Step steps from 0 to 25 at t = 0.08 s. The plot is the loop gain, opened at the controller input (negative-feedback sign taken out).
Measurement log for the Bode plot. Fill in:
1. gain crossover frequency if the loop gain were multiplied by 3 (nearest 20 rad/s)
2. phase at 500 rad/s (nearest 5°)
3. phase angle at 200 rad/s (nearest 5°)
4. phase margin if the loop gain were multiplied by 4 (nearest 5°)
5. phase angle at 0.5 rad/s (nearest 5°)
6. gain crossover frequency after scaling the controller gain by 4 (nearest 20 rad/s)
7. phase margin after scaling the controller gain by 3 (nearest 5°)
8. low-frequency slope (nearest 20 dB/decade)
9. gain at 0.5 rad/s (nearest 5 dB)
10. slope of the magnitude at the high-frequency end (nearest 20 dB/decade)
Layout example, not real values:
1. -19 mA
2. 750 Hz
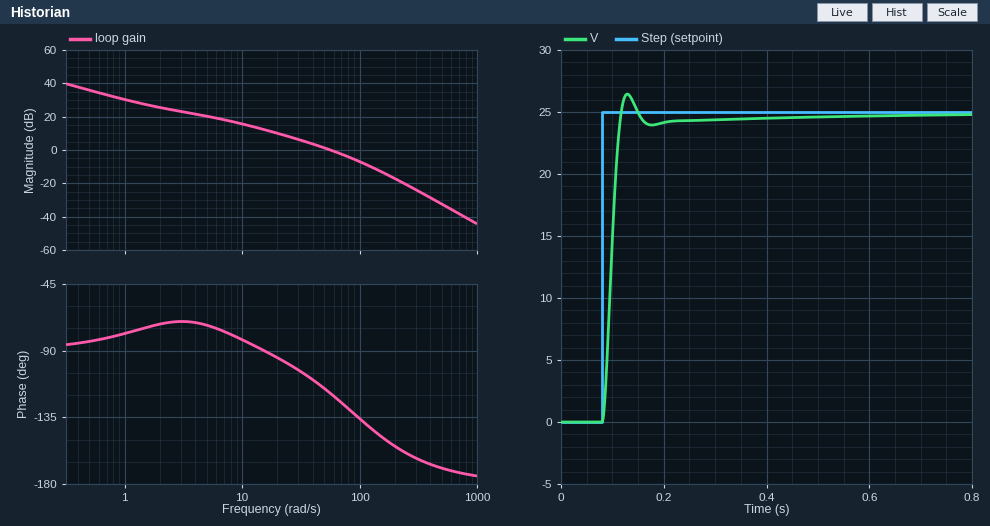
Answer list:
1. 120 rad/s
2. -170°
3. -155°
4. 35°
5. -85°
6. 140 rad/s
7. 40°
8. -20 dB/decade
9. 35 dB
10. -40 dB/decade
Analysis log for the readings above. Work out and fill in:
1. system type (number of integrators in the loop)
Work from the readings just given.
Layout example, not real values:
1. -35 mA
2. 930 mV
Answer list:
1. 1
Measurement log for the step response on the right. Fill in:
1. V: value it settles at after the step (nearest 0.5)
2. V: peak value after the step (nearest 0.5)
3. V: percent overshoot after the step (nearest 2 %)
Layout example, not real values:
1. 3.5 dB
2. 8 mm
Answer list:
1. 25.0
2. 26.5
3. 6 %
